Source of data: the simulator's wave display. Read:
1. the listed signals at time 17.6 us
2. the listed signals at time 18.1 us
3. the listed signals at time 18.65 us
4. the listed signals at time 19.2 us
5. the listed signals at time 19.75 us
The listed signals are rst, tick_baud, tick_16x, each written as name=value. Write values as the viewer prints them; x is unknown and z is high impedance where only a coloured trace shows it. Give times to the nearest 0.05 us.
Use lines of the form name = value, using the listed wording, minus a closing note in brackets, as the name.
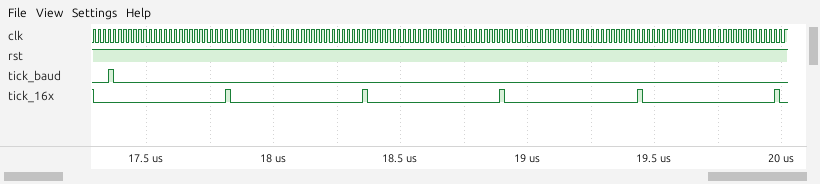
the listed signals at time 17.6 us = rst=1, tick_baud=0, tick_16x=0
the listed signals at time 18.1 us = rst=1, tick_baud=0, tick_16x=0
the listed signals at time 18.65 us = rst=1, tick_baud=0, tick_16x=0
the listed signals at time 19.2 us = rst=1, tick_baud=0, tick_16x=0
the listed signals at time 19.75 us = rst=1, tick_baud=0, tick_16x=0
